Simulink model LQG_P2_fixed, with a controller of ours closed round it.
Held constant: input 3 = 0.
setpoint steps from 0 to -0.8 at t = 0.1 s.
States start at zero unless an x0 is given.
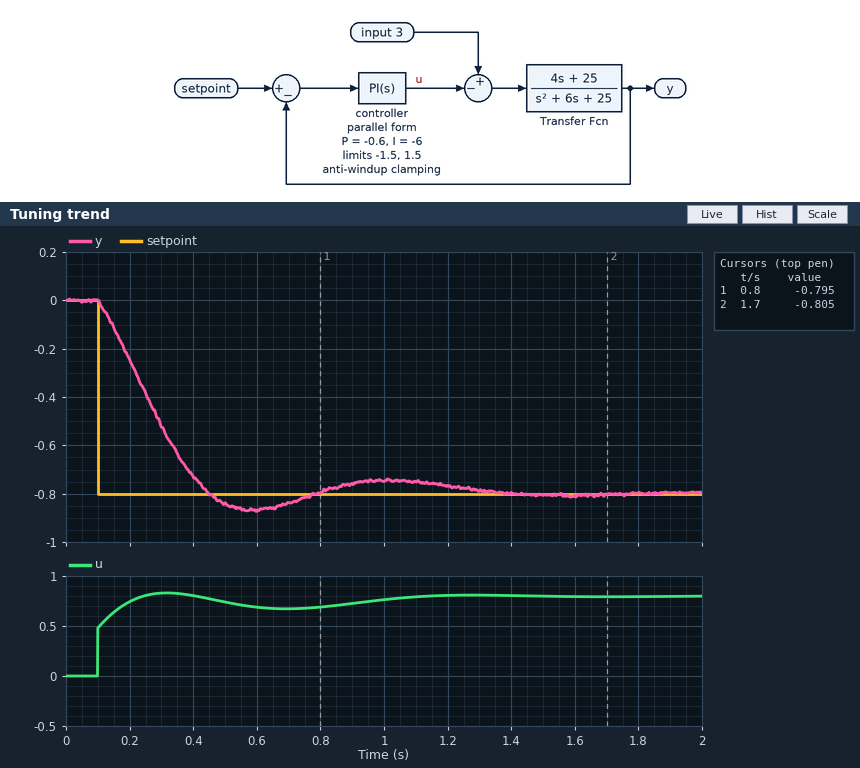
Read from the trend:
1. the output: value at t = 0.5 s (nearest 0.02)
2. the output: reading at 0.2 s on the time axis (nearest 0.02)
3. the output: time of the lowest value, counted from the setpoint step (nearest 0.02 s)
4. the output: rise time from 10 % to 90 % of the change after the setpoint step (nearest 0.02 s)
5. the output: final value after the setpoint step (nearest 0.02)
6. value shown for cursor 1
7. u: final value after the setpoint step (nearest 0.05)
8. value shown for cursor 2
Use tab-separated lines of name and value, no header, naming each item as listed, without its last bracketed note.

the output: value at t = 0.5 s	-0.84
the output: reading at 0.2 s on the time axis	-0.24
the output: time of the lowest value, counted from the setpoint step	0.48 s
the output: rise time from 10 % to 90 % of the change after the setpoint step	0.26 s
the output: final value after the setpoint step	-0.80
value shown for cursor 1	-0.795
u: final value after the setpoint step	0.80
value shown for cursor 2	-0.805
